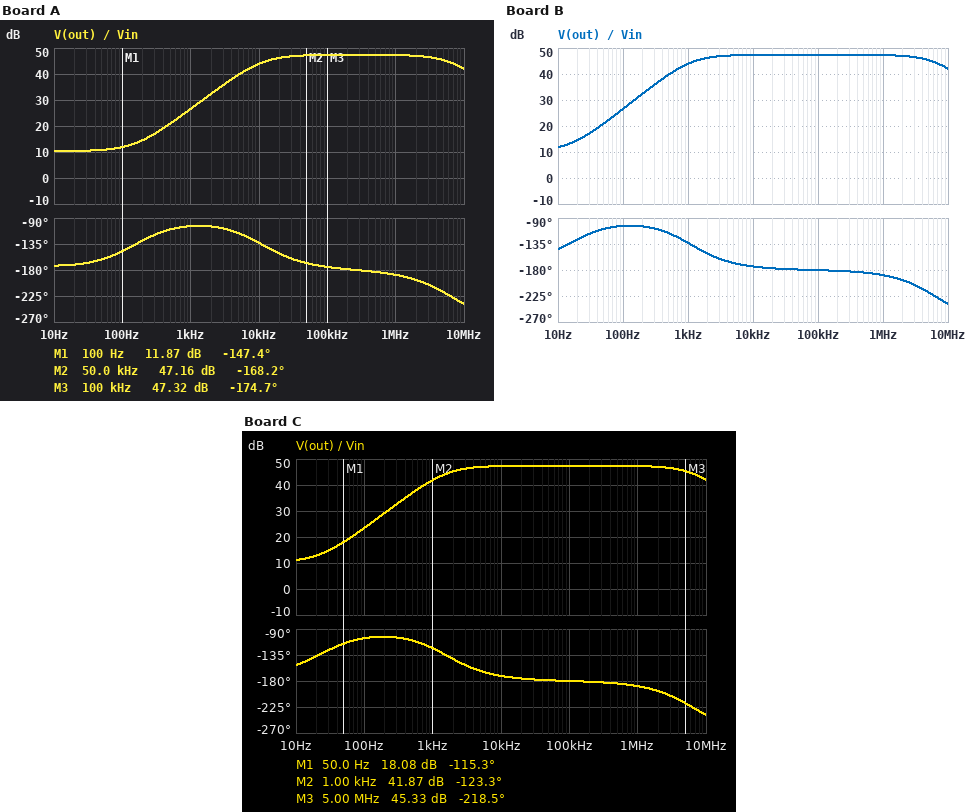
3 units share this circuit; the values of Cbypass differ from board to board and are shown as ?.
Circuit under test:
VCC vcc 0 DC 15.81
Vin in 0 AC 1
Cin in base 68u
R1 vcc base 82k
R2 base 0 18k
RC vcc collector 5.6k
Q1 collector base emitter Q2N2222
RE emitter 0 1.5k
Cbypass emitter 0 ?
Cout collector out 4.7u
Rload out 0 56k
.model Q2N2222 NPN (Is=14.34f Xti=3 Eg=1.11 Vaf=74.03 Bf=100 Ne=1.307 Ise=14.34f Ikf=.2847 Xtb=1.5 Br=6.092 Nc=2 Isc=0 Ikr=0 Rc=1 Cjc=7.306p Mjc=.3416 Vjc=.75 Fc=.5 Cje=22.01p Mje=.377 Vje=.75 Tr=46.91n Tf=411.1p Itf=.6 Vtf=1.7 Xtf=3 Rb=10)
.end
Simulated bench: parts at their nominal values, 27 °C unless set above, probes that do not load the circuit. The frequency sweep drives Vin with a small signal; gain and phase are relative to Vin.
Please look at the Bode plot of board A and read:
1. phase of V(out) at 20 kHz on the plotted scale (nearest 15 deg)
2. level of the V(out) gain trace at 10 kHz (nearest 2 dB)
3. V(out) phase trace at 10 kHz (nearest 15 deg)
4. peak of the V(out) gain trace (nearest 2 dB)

-150 deg
44 dB
-135 deg
48 dB
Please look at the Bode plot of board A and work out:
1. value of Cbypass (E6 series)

680 nF
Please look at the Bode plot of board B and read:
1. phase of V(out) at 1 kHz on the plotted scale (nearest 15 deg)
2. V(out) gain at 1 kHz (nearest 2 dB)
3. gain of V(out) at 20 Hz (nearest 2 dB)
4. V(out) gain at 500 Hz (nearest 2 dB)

-135 deg
44 dB
14 dB
40 dB
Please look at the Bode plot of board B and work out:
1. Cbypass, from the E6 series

6.8 µF
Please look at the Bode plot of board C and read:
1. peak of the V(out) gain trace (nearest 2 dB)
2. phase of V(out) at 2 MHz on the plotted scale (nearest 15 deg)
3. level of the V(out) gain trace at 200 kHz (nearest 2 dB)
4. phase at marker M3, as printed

48 dB
-195 deg
48 dB
-218.5 deg
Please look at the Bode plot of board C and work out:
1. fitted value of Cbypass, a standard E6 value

4.7 µF
